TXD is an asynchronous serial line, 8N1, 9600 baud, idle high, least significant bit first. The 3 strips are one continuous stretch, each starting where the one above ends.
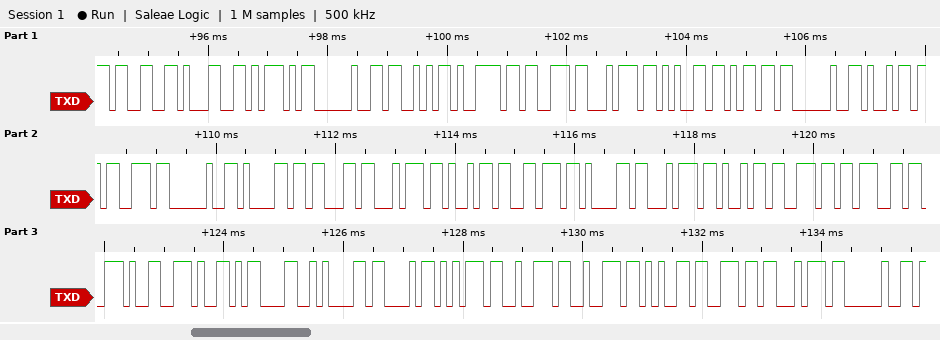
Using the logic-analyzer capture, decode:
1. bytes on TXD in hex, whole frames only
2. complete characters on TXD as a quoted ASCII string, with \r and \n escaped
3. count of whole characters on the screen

33 31 5D 20 53 79 73 74 65 6D 20 69 73 20 61 63 74 69 76 61 74 69 6E 67 2E 2E 0D 0A 43 75 72 72 65 6E 74 20
"31] System is activating..\r\nCurrent "
36
